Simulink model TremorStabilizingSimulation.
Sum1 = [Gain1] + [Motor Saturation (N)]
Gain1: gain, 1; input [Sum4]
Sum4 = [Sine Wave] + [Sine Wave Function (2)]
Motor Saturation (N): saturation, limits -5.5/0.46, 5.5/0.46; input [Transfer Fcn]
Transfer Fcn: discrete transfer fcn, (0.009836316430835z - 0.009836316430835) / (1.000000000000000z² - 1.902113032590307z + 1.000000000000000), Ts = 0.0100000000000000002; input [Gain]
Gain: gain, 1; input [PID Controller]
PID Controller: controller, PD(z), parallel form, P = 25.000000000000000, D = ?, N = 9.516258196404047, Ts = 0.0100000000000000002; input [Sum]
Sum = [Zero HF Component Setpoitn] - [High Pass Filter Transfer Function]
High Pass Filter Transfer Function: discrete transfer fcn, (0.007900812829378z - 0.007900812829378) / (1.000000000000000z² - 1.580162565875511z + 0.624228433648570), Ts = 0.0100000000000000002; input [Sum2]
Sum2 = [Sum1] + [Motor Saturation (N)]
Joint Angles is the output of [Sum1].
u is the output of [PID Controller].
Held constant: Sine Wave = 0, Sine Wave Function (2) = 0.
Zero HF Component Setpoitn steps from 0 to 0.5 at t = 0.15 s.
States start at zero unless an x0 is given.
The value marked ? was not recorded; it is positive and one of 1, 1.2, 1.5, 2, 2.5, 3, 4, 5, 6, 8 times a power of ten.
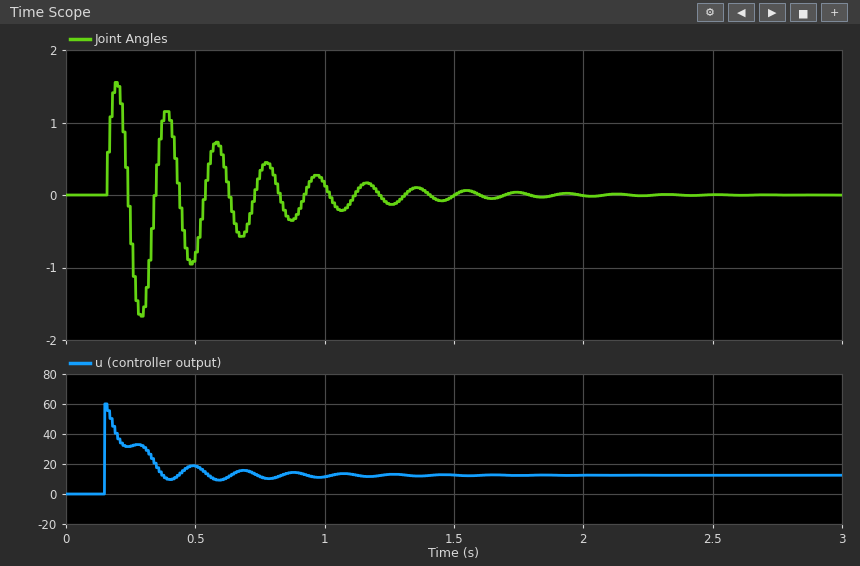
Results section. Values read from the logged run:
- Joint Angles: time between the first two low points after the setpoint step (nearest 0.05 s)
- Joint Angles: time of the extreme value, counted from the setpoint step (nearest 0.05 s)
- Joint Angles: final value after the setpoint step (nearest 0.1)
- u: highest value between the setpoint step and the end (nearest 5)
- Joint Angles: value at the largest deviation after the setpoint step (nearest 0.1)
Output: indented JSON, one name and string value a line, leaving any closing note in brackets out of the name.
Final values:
{
  "Joint Angles: time between the first two low points after the setpoint step": "0.20 s",
  "Joint Angles: time of the extreme value, counted from the setpoint step": "0.15 s",
  "Joint Angles: final value after the setpoint step": "0.0",
  "u: highest value between the setpoint step and the end": "60",
  "Joint Angles: value at the largest deviation after the setpoint step": "-1.7"
}
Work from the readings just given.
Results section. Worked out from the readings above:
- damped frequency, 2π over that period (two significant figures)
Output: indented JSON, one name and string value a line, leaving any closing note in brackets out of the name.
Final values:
{
  "damped frequency, 2π over that period": "31 rad/s"
}
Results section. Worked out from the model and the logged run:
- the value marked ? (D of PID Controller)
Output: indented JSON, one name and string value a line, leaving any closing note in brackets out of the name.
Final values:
{
  "the value marked ?": "10"
}
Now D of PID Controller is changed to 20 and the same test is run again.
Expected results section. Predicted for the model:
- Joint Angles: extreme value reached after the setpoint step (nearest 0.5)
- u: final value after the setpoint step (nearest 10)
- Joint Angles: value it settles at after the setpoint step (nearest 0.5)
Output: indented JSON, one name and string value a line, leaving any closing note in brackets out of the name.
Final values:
{
  "Joint Angles: extreme value reached after the setpoint step": "2.5",
  "u: final value after the setpoint step": "10",
  "Joint Angles: value it settles at after the setpoint step": "0.0"
}
